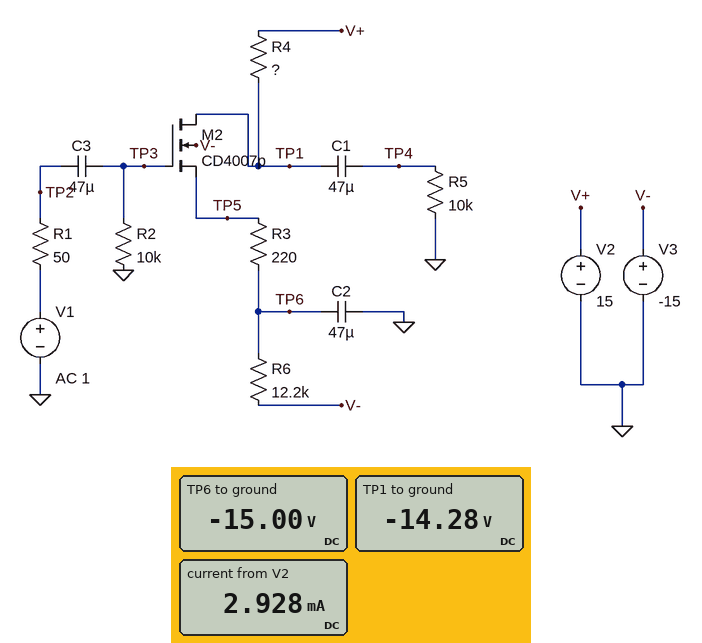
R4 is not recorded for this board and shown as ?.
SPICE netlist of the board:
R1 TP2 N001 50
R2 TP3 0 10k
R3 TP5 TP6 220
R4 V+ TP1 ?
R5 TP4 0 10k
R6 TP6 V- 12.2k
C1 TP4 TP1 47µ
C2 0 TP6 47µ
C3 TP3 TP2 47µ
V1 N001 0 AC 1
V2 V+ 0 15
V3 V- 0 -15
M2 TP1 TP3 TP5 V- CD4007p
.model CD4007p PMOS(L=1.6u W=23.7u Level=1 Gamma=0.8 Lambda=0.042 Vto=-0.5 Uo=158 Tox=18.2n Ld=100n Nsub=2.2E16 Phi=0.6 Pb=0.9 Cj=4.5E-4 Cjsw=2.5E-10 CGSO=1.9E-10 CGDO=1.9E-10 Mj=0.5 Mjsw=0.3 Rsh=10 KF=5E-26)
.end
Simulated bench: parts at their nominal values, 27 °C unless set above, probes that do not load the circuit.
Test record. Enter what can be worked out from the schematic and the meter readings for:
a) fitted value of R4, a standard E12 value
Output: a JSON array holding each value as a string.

["10 kΩ"]
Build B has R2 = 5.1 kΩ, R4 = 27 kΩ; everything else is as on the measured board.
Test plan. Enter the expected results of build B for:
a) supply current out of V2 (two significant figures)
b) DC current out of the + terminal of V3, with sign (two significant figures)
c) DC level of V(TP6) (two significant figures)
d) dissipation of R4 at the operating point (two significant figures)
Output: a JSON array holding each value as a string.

["1.1 mA", "-1.1 mA", "-15 V", "32 mW"]
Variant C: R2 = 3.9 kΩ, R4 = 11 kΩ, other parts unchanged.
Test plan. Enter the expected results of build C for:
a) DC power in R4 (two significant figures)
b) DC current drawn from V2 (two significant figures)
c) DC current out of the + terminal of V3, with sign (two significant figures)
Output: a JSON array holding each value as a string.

["78 mW", "2.7 mA", "-2.7 mA"]
